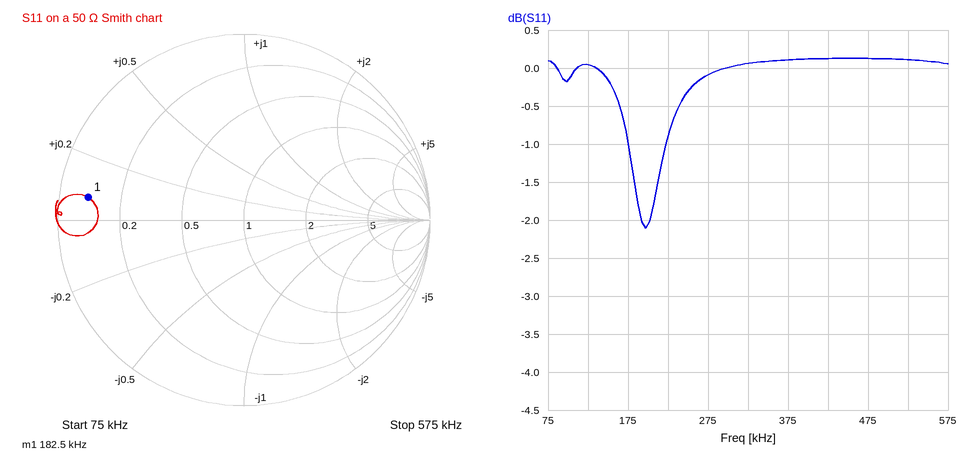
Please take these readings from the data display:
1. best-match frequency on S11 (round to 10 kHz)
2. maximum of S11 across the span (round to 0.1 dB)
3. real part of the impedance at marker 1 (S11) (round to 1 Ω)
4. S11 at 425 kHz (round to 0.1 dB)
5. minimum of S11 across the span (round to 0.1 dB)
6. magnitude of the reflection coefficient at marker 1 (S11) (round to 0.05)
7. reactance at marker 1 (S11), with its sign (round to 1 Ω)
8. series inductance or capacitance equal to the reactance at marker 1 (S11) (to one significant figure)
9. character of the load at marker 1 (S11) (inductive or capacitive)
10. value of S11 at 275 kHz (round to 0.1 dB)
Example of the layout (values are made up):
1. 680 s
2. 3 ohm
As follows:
1. 200 kHz
2. 0.1 dB
3. 4 Ω
4. 0.1 dB
5. -2.1 dB
6. 0.85
7. +4 Ω
8. 3 µH
9. inductive
10. -0.1 dB
